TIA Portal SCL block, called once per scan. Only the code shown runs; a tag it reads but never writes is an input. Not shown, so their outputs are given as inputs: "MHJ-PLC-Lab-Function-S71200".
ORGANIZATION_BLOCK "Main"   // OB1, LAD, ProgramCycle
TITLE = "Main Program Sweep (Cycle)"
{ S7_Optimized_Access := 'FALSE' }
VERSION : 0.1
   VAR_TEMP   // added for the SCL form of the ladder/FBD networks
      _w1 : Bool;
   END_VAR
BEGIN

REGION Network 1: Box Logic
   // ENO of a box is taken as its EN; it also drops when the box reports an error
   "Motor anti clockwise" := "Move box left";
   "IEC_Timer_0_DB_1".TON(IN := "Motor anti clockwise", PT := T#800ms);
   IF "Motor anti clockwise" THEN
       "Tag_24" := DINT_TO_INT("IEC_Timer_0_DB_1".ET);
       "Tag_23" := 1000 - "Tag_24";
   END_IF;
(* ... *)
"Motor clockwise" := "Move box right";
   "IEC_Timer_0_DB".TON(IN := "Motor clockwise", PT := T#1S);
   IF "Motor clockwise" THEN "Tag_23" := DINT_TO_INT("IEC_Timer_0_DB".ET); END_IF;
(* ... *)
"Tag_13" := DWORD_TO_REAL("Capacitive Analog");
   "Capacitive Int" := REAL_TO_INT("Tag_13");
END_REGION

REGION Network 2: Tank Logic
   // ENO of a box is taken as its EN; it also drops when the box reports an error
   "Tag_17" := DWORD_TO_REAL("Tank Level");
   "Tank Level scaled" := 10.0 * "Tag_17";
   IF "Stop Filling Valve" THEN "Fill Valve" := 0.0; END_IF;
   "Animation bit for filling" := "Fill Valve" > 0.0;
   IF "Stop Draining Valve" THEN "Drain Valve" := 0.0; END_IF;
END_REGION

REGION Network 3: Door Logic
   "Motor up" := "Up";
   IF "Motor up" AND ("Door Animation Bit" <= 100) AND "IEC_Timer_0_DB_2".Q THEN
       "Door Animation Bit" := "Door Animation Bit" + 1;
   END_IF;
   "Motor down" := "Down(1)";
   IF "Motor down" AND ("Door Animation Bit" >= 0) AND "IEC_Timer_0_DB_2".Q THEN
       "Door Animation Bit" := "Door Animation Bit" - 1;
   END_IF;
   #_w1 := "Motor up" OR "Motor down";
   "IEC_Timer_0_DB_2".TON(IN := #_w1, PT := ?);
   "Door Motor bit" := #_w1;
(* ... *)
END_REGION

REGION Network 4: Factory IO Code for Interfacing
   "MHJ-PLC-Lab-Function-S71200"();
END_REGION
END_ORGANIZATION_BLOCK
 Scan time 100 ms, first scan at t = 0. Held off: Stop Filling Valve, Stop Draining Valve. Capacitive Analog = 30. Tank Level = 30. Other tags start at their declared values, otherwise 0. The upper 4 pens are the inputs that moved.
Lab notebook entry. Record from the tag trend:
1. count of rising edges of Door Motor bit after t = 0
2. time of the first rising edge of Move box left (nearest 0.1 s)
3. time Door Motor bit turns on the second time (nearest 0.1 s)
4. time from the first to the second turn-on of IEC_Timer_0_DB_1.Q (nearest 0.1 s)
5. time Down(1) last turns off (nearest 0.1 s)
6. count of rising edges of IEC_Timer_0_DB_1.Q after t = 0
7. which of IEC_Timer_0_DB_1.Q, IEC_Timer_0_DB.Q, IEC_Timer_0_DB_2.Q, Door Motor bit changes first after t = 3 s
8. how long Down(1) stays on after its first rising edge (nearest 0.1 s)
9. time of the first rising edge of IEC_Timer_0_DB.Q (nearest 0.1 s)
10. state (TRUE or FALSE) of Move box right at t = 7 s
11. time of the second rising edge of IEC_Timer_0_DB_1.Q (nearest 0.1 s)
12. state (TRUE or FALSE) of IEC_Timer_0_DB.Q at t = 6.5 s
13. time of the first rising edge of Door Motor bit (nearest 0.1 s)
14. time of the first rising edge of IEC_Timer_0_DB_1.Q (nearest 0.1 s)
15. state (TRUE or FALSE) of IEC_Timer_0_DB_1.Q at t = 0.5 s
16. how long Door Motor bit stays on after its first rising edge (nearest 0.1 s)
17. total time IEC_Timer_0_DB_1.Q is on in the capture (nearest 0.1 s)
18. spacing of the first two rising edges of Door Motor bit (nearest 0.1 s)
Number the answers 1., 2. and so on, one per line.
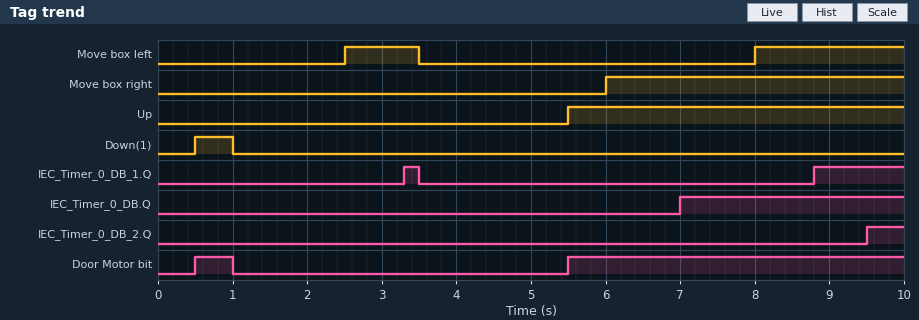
1. 2
2. 2.5 s
3. 5.5 s
4. 5.5 s
5. 1.0 s
6. 2
7. IEC_Timer_0_DB_1.Q
8. 0.5 s
9. 7.0 s
10. TRUE
11. 8.8 s
12. FALSE
13. 0.5 s
14. 3.3 s
15. FALSE
16. 0.5 s
17. 1.4 s
18. 5.0 s
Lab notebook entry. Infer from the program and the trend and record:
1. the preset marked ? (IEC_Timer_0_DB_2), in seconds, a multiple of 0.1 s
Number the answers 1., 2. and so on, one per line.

1. 4.0 s
